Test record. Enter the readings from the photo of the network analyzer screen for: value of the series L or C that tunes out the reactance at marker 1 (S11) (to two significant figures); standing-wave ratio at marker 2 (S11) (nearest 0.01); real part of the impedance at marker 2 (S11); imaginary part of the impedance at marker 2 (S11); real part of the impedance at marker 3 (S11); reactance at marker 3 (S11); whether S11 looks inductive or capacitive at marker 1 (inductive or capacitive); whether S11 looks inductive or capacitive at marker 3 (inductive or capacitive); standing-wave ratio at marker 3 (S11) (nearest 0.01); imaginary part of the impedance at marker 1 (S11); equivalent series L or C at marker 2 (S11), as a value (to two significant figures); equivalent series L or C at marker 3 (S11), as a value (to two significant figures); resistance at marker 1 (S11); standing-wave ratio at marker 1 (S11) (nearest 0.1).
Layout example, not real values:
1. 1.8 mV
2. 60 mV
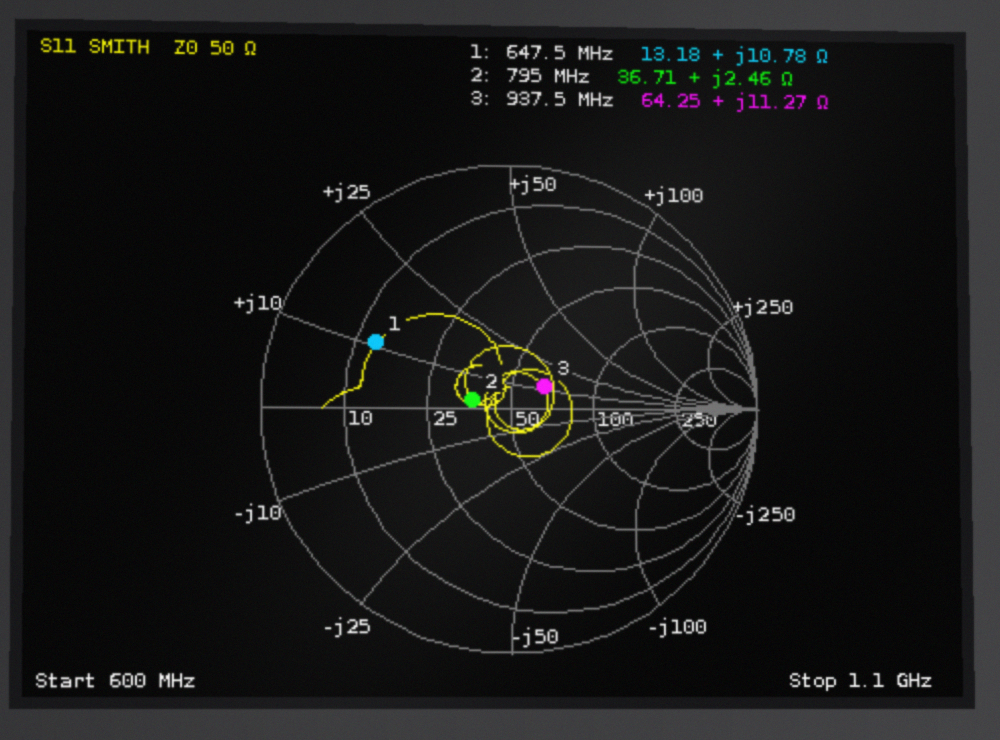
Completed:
1. 23 pF
2. 1.37
3. 36.71 Ω
4. +2.46 Ω
5. 64.25 Ω
6. +11.27 Ω
7. inductive
8. inductive
9. 1.38
10. +10.78 Ω
11. 490 pH
12. 1.9 nH
13. 13.18 Ω
14. 4.0
